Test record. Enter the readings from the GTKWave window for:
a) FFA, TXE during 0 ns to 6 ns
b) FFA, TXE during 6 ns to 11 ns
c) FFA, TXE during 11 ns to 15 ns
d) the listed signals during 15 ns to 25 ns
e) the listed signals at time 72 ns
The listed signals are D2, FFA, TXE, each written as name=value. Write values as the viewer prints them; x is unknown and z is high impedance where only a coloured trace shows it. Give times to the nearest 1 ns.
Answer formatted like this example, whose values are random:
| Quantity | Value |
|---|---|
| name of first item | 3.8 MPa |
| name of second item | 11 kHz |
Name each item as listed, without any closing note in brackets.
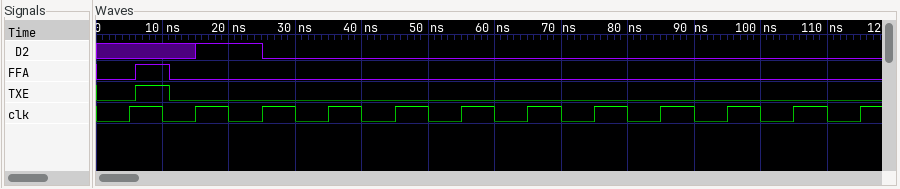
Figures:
| Quantity | Value |
|---|---|
| FFA, TXE during 0 ns to 6 ns | FFA=0, TXE=0 |
| FFA, TXE during 6 ns to 11 ns | FFA=1, TXE=1 |
| FFA, TXE during 11 ns to 15 ns | FFA=0, TXE=0 |
| the listed signals during 15 ns to 25 ns | D2=1, FFA=0, TXE=0 |
| the listed signals at time 72 ns | D2=0, FFA=0, TXE=0 |
